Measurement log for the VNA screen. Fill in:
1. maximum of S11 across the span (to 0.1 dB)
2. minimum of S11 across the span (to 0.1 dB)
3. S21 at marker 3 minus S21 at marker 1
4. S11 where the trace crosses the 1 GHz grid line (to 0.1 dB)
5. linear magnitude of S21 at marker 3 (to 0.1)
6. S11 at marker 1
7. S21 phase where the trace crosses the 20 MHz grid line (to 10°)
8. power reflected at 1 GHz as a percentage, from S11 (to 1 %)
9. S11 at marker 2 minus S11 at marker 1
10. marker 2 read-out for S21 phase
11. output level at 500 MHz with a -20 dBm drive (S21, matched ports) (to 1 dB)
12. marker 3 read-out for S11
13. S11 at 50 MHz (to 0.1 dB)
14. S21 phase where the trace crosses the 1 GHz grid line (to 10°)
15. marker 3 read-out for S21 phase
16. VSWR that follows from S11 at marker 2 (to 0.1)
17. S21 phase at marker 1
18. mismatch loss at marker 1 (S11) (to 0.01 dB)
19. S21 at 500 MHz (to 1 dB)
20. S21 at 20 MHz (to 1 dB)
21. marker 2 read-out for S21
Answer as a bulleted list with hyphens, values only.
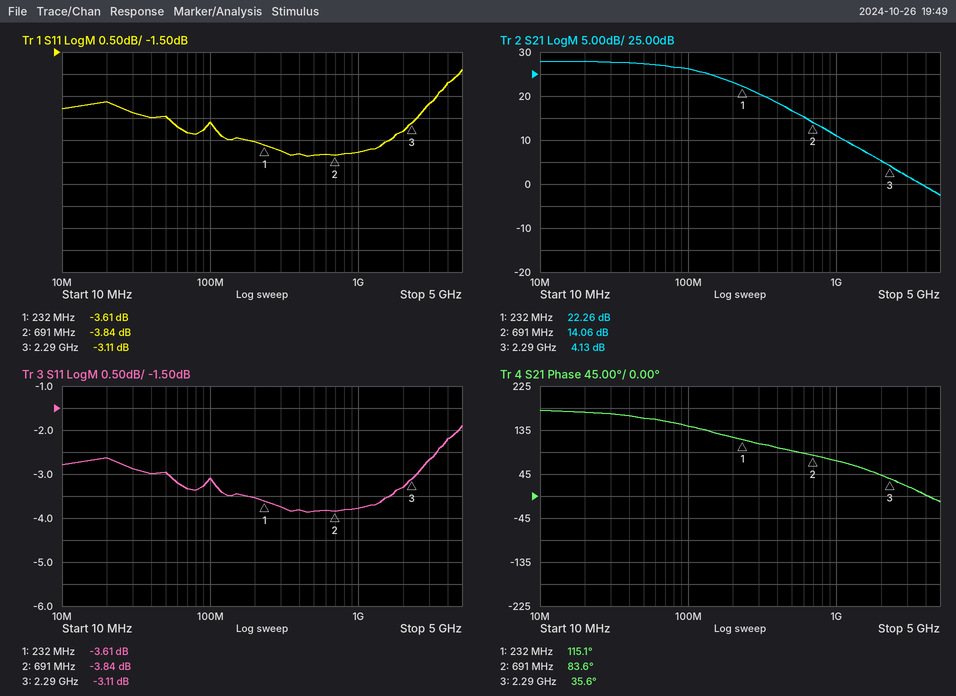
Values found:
- -1.9 dB
- -3.9 dB
- -18.13 dB
- -3.8 dB
- 1.6
- -3.61 dB
- 170°
- 42 %
- -0.23 dB
- 83.6°
- -3 dBm
- -3.11 dB
- -3.0 dB
- 70°
- 35.6°
- 4.6
- 115.1°
- 2.48 dB
- 17 dB
- 28 dB
- 14.06 dB
